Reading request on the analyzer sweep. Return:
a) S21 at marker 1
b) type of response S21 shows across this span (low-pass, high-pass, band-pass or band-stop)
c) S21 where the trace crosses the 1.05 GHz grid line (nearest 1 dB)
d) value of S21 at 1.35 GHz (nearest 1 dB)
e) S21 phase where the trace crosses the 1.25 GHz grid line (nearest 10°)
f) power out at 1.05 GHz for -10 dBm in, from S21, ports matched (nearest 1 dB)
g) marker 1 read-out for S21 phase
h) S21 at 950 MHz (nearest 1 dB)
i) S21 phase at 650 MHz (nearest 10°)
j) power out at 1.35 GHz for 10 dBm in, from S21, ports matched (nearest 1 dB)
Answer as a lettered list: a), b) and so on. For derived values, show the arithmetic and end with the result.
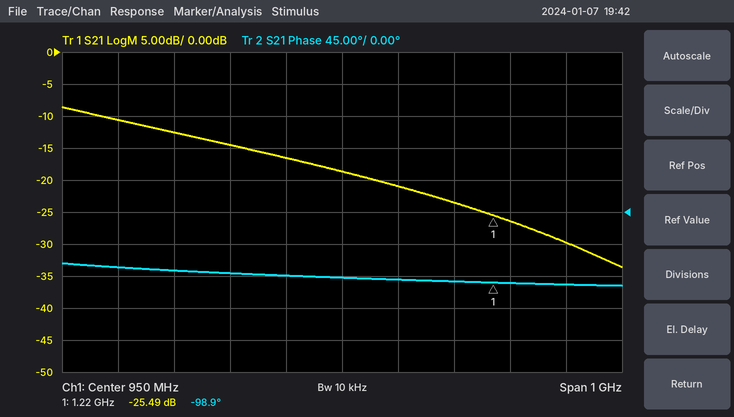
a) -25.49 dB
b) low-pass
c) -21 dB
d) -30 dB
e) -100°
f) -10 dBm + (-21 dB) = -31 dBm
g) -98.9°
h) -19 dB
i) -80°
j) 10 dBm + (-30 dB) = -20 dBm
